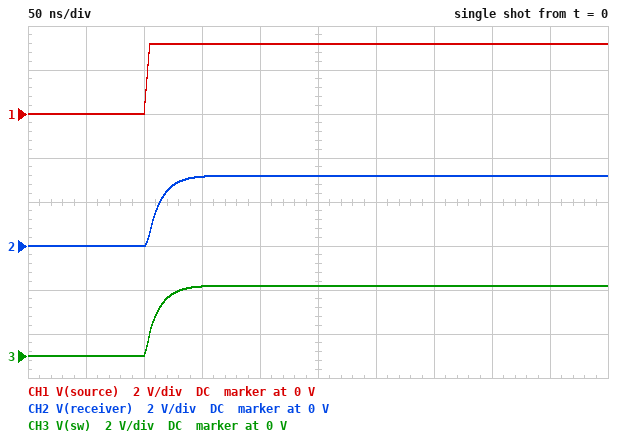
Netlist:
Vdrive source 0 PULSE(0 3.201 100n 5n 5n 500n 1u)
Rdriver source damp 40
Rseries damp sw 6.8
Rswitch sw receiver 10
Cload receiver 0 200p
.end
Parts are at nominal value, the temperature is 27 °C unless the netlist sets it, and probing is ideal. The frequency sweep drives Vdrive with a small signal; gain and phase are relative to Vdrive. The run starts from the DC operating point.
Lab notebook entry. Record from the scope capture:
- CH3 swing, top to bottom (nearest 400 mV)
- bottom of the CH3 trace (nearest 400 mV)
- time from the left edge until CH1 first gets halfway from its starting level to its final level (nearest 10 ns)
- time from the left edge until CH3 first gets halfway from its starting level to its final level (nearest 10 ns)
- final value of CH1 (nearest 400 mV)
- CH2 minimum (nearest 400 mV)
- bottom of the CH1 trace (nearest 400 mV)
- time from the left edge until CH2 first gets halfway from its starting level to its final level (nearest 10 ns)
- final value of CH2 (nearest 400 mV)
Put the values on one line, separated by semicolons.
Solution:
3.2 V; 0 V; 100 ns; 110 ns; 3.2 V; 0 V; 0 V; 110 ns; 3.2 V
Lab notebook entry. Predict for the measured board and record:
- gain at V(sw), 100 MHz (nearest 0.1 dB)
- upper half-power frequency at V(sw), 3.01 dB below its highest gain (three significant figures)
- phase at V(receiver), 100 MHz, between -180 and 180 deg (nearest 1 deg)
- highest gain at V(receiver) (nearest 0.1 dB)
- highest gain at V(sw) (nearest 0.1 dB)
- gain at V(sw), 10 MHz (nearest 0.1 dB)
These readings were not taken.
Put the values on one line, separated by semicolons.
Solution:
-13.0 dB; 14.5 MHz; -82 deg; 0 dB; 0 dB; -1.7 dB
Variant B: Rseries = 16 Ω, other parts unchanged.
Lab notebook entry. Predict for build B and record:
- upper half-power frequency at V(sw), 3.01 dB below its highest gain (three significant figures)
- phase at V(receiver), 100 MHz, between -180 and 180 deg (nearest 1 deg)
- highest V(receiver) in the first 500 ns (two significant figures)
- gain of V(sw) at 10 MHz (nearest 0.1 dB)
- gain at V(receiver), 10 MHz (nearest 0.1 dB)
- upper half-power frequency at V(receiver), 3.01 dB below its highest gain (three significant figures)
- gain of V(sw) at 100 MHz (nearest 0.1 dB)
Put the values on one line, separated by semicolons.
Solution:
12.3 MHz; -83 deg; 3.2 V; -2.2 dB; -2.3 dB; 12.1 MHz; -14.3 dB
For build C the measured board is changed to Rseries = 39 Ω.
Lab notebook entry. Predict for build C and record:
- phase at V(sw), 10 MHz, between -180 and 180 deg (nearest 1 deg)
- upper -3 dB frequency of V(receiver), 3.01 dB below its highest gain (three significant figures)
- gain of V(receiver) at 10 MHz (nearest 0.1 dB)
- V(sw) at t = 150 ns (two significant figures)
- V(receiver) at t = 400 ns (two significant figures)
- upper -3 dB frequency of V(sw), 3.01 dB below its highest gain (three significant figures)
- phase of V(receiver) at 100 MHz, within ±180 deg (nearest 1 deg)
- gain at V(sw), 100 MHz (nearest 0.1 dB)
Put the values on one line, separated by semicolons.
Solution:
-41 deg; 8.94 MHz; -3.5 dB; 3.0 V; 3.2 V; 9.06 MHz; -85 deg; -16.9 dB
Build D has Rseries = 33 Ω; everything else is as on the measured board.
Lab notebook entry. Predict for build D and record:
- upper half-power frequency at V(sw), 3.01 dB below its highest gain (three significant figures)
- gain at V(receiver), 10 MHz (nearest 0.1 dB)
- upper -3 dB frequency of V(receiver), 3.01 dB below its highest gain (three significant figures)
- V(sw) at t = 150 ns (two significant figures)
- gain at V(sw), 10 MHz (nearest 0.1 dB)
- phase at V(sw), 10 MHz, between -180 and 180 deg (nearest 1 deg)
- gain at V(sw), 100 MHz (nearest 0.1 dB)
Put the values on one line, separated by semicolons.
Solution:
9.73 MHz; -3.2 dB; 9.59 MHz; 3.0 V; -3.1 dB; -39 deg; -16.3 dB
